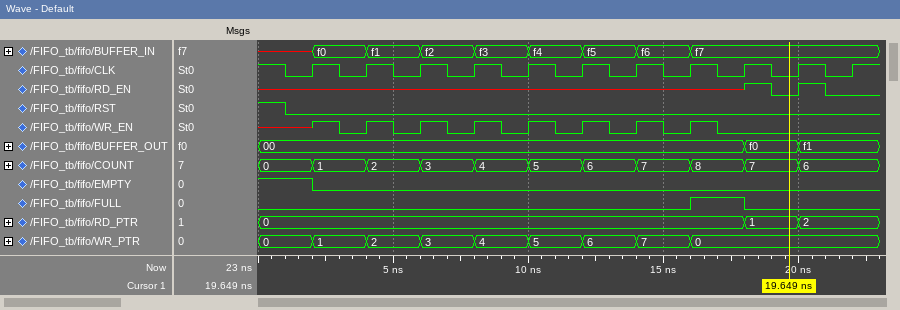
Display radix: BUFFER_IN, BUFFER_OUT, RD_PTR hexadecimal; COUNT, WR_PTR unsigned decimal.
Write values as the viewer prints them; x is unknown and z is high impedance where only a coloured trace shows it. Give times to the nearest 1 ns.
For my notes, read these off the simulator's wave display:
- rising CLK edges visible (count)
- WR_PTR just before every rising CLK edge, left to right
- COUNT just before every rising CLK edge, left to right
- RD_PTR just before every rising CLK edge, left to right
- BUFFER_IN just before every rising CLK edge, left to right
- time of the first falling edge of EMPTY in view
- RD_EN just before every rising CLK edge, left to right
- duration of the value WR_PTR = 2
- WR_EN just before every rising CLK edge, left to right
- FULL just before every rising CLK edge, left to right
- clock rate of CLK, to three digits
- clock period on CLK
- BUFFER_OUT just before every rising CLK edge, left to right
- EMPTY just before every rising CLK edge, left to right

11
0, 1, 2, 3, 4, 5, 6, 7, 0, 0, 0
0, 1, 2, 3, 4, 5, 6, 7, 8, 7, 6
0, 0, 0, 0, 0, 0, 0, 0, 0, 1, 2
x, f0, f1, f2, f3, f4, f5, f6, f7, f7, f7
2 ns
x x x x x x x x x 0 0
2 ns
x 0 0 0 0 0 0 0 0 0 0
0 0 0 0 0 0 0 0 1 0 0
500 MHz
2 ns
00, 00, 00, 00, 00, 00, 00, 00, 00, f0, f1
1 0 0 0 0 0 0 0 0 0 0
